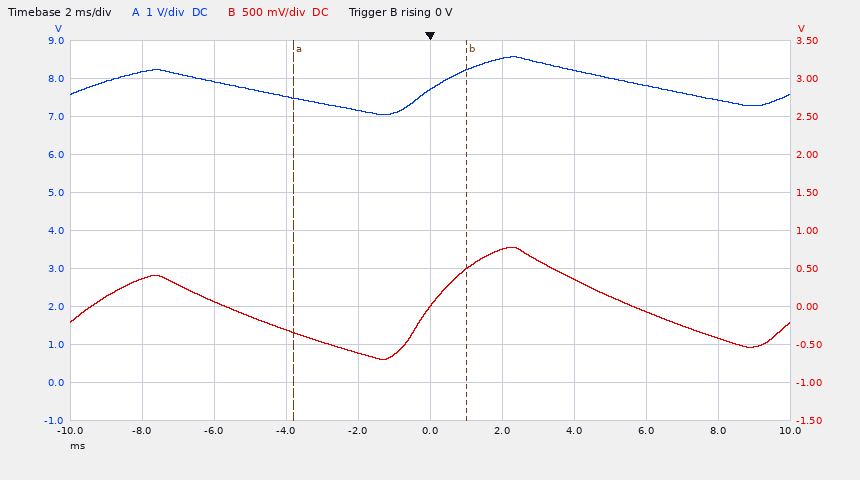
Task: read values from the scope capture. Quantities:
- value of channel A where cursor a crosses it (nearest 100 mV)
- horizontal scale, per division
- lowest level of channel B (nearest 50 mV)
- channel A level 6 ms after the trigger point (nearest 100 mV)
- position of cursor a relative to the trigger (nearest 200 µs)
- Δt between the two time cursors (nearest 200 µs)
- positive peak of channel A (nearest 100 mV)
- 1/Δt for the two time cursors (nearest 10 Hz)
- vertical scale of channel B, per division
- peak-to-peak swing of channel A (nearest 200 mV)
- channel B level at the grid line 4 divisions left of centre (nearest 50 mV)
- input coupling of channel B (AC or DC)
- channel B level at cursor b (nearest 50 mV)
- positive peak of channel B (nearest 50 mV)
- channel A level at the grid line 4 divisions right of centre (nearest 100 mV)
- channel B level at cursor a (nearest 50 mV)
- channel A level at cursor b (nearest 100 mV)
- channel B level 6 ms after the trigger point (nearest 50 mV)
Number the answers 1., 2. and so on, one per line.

1. 7.5 V
2. 2 ms
3. -700 mV
4. 7.8 V
5. -3.8 ms
6. 4.8 ms
7. 8.6 V
8. 210 Hz
9. 500 mV
10. 1.6 V
11. 350 mV
12. DC
13. 500 mV
14. 800 mV
15. 7.4 V
16. -350 mV
17. 8.2 V
18. -50 mV
